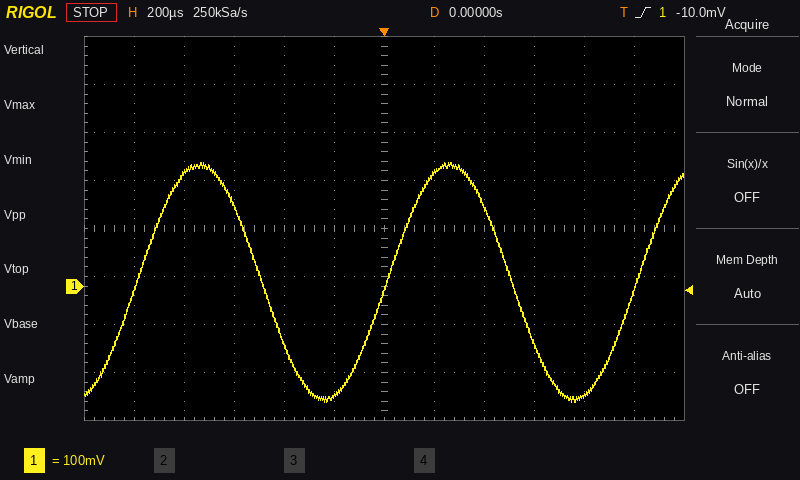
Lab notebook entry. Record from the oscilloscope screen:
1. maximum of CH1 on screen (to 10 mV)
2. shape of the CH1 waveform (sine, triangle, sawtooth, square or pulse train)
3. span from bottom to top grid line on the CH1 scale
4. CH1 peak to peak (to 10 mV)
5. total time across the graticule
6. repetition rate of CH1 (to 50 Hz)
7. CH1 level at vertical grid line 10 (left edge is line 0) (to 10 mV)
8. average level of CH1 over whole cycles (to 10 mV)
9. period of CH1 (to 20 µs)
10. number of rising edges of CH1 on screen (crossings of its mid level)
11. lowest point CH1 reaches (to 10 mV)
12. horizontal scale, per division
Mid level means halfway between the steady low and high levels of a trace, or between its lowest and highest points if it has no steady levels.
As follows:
260 mV
sine
800 mV
500 mV
2.4 ms
1.00 kHz
-230 mV
10 mV
1.00 ms
3
-240 mV
200 µs
